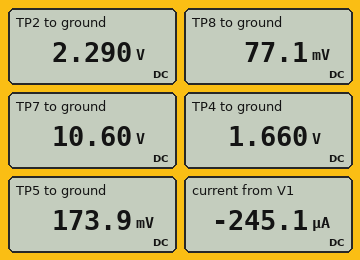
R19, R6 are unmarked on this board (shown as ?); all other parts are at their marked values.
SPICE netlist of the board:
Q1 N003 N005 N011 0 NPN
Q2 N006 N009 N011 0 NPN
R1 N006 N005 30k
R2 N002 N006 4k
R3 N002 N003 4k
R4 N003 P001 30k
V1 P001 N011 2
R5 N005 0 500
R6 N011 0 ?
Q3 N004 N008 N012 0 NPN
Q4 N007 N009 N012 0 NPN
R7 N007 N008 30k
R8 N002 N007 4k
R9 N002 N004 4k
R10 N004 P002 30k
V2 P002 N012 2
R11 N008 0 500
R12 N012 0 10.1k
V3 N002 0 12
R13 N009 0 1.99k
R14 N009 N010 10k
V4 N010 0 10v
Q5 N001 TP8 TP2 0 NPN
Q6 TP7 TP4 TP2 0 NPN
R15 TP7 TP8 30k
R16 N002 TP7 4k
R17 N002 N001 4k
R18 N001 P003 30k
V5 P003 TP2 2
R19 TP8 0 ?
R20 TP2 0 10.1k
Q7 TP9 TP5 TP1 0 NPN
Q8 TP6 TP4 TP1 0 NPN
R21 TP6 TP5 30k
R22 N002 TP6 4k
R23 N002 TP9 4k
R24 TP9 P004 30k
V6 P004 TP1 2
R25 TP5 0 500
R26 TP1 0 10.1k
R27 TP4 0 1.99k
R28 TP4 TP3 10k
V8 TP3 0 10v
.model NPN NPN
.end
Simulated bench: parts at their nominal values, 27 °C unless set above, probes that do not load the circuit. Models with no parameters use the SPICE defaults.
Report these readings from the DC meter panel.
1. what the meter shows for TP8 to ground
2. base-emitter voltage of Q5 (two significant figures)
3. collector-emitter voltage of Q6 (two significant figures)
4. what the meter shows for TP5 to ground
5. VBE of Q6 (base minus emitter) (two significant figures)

77.1 mV
-2.2 V
8.3 V
173.9 mV
-630 mV
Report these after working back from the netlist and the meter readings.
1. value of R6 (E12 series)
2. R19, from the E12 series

6.8 kΩ
220 Ω
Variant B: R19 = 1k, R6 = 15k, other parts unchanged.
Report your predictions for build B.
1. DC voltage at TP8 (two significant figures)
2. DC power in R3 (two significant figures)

340 mV
170 µW
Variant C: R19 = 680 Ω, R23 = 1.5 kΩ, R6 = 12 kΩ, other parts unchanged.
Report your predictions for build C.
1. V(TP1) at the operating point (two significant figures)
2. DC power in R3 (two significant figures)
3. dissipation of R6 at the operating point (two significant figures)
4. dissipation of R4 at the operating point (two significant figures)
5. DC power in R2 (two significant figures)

2.4 V
190 µW
570 µW
1.4 mW
480 µW
